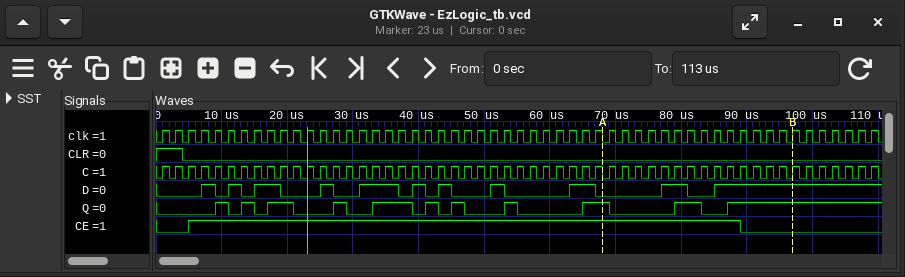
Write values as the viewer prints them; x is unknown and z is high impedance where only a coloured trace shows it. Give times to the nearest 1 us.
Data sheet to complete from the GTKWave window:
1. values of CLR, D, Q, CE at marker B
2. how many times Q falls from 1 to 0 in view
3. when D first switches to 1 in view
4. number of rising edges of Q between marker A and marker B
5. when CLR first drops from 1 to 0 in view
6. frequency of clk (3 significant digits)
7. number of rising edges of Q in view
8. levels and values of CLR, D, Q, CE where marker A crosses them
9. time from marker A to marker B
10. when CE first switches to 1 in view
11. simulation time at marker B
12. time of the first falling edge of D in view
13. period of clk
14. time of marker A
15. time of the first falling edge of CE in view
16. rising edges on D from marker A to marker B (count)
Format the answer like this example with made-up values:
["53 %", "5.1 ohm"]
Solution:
["CLR=0, D=1, Q=1, CE=0", "10", "7 us", "2", "4 us", "500 kHz", "11", "CLR=0, D=0, Q=1, CE=1", "29 us", "5 us", "97 us", "9 us", "2 us", "68 us", "89 us", "2"]
